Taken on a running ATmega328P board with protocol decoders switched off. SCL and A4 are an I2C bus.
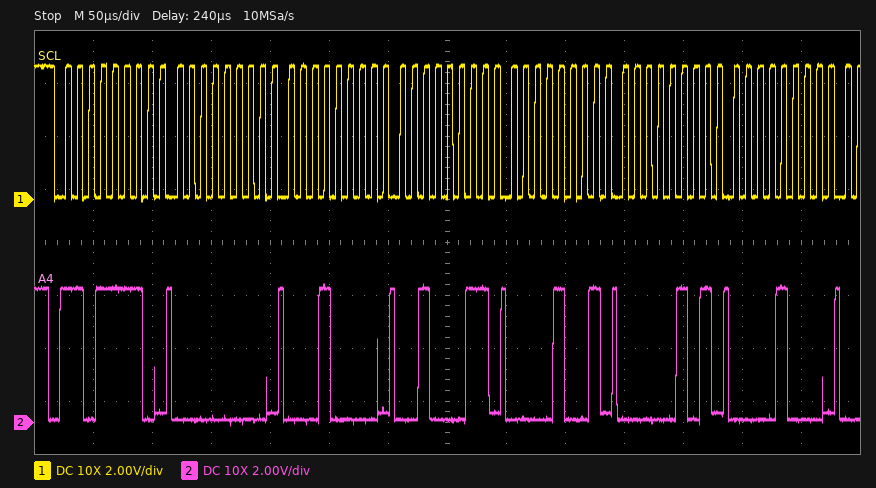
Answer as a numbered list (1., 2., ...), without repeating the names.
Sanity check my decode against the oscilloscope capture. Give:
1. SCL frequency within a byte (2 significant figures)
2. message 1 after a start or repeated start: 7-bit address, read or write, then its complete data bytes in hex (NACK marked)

1. 100 kHz
2. 0x6F write: 00 10 23 09 05 08
